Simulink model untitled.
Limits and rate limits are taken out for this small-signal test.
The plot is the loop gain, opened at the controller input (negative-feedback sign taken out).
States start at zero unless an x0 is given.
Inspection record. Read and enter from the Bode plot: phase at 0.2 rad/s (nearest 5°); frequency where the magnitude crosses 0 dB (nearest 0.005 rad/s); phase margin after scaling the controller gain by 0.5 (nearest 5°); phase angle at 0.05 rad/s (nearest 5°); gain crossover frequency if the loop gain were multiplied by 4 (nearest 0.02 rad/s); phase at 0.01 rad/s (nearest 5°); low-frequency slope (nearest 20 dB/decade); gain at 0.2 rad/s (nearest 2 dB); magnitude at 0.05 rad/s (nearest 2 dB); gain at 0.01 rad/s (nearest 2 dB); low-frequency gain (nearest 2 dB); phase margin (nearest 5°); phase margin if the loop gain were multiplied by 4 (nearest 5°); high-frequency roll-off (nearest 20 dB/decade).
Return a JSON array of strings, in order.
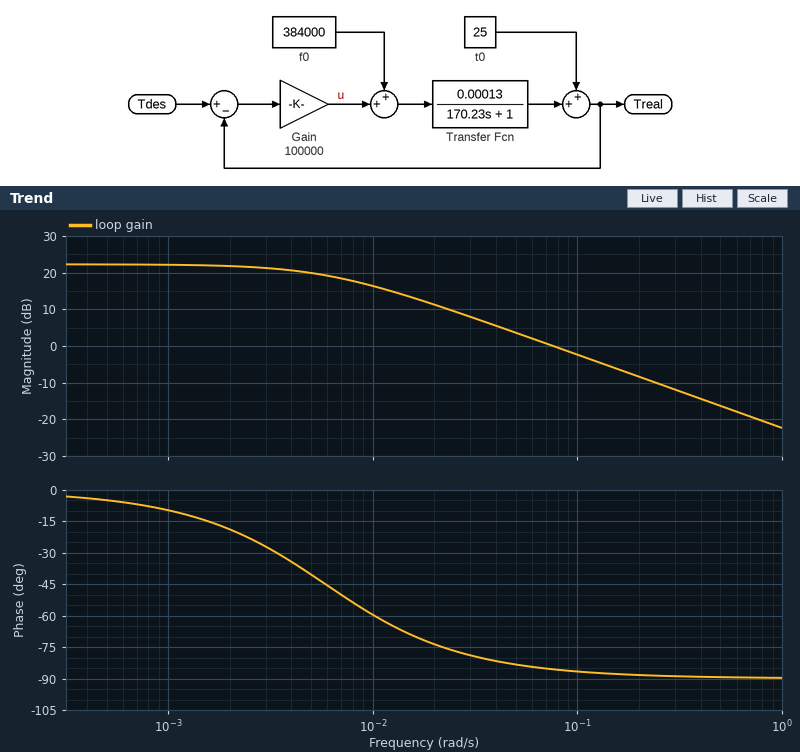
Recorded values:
["-90°", "0.075 rad/s", "100°", "-85°", "0.30 rad/s", "-60°", "0 dB/decade", "-8 dB", "4 dB", "16 dB", "22 dB", "95°", "90°", "-20 dB/decade"]
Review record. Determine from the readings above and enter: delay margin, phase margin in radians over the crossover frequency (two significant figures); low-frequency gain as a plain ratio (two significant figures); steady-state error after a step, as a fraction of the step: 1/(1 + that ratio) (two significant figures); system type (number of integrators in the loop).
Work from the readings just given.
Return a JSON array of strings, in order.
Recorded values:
["22 s", "13", "0.071", "0"]
